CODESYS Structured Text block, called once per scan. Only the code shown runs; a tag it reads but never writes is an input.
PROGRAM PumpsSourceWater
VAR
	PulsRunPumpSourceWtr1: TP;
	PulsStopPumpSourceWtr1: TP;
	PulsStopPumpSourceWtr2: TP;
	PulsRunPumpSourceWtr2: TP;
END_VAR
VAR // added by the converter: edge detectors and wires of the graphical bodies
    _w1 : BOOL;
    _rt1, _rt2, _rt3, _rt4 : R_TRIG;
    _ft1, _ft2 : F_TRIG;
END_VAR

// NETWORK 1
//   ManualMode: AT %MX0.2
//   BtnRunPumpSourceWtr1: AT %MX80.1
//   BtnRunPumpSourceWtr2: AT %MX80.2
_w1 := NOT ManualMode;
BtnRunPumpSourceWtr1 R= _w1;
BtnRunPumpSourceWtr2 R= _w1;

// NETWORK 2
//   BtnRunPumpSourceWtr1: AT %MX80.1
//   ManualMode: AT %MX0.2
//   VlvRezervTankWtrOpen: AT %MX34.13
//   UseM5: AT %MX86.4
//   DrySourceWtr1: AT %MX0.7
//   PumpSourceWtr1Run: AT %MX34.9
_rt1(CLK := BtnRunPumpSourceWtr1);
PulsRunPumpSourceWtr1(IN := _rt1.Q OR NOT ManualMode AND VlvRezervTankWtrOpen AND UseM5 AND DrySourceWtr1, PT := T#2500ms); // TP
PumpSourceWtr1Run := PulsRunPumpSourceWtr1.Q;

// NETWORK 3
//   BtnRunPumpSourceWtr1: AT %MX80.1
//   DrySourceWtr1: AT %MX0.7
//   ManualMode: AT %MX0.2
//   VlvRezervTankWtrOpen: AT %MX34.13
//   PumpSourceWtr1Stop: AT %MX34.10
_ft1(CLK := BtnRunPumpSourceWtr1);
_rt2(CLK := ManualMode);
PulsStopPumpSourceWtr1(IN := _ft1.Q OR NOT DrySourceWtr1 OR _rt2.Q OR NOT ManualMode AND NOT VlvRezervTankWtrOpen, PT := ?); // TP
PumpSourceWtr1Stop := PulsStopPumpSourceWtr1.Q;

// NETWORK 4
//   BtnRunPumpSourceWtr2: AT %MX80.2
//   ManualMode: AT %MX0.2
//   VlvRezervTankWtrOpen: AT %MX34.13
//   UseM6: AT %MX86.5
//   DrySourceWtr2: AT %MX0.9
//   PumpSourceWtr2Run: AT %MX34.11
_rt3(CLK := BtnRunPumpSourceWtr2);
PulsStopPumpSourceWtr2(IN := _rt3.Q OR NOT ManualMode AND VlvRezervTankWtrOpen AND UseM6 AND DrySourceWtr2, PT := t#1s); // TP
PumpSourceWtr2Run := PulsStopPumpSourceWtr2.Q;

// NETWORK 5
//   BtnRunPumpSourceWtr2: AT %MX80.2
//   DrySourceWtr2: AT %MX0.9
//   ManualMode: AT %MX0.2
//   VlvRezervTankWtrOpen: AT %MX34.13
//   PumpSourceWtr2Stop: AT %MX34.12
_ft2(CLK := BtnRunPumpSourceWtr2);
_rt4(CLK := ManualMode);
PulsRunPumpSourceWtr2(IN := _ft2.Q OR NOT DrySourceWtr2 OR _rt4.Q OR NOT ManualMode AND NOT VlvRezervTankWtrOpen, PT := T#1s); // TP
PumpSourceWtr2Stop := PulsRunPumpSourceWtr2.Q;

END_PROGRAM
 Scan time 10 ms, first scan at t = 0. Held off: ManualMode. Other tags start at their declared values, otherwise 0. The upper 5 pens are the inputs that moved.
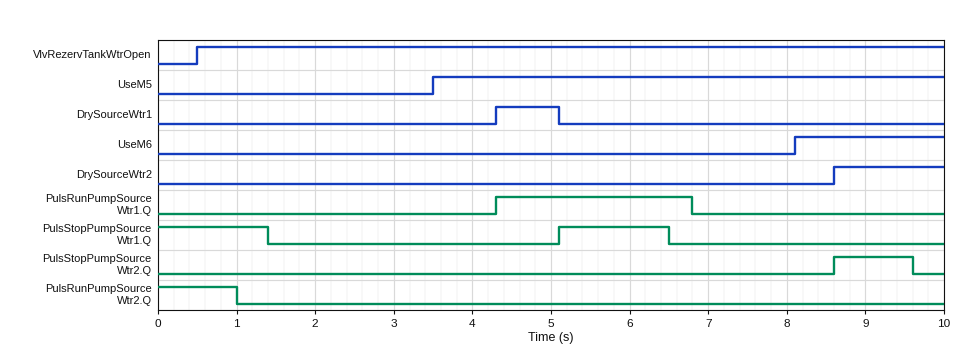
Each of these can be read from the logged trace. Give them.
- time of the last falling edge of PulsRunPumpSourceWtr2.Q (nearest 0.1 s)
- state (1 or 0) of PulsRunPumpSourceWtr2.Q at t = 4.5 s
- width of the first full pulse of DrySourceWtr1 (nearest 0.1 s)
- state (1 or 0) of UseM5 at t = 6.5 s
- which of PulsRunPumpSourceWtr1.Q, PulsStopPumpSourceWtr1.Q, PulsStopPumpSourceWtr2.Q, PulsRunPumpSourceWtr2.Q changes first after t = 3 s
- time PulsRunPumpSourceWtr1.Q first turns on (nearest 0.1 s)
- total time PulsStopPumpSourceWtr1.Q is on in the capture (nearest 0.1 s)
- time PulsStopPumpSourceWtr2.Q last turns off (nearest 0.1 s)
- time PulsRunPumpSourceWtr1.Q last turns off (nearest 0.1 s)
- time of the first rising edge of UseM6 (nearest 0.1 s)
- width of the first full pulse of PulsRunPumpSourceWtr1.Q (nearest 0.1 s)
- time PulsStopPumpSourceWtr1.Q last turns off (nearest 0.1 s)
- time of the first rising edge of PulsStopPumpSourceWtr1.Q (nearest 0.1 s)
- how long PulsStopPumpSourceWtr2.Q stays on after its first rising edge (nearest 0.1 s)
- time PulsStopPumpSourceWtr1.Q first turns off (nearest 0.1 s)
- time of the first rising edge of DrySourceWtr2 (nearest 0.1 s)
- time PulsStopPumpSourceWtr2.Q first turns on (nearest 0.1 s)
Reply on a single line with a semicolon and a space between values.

1.0 s; 0; 0.8 s; 1; PulsRunPumpSourceWtr1.Q; 4.3 s; 2.8 s; 9.6 s; 6.8 s; 8.1 s; 2.5 s; 6.5 s; 5.1 s; 1.0 s; 1.4 s; 8.6 s; 8.6 s
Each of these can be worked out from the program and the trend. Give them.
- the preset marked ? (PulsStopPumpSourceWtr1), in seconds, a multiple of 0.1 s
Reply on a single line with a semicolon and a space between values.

1.4 s
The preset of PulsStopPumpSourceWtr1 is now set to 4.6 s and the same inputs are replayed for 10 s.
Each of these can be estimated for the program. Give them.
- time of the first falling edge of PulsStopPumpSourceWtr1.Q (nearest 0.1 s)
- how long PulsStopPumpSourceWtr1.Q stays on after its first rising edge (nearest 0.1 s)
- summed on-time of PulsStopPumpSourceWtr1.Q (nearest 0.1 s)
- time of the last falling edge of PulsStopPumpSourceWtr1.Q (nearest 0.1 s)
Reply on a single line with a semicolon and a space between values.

4.6 s; 4.6 s; 9.2 s; 9.7 s
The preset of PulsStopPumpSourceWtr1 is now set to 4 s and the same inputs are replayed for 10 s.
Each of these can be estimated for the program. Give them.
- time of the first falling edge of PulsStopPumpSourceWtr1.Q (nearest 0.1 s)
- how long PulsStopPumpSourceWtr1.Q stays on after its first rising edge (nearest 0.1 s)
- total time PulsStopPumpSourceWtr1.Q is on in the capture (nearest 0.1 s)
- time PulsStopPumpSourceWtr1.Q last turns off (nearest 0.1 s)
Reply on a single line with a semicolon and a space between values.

4.0 s; 4.0 s; 8.0 s; 9.1 s
